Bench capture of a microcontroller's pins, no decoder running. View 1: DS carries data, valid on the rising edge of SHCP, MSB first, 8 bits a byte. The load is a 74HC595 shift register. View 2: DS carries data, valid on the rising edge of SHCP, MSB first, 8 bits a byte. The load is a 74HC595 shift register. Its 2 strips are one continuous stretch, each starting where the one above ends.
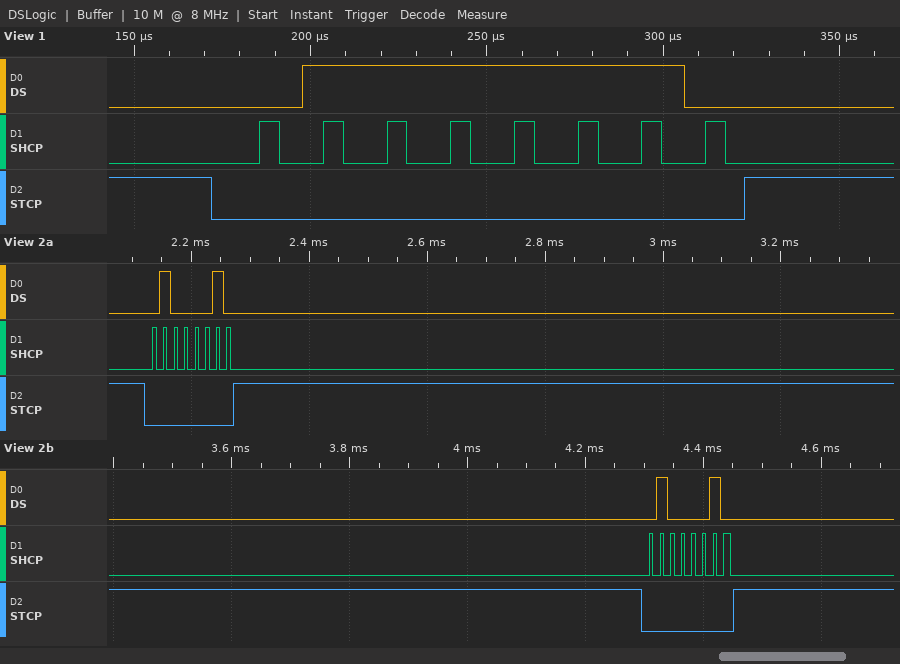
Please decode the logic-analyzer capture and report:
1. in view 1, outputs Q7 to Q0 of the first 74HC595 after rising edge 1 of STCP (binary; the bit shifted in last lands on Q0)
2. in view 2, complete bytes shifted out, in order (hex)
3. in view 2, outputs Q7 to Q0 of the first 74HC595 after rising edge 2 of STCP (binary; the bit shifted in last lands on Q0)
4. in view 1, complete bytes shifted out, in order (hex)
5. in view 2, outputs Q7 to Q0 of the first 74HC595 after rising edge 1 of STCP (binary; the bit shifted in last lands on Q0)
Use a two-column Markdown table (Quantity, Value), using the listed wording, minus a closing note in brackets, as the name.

| Quantity | Value |
|---|---|
| in view 1, outputs Q7 to Q0 of the first 74HC595 after rising edge 1 of STCP | 01111110 |
| in view 2, complete bytes shifted out, in order | 0x42 0x42 |
| in view 2, outputs Q7 to Q0 of the first 74HC595 after rising edge 2 of STCP | 01000010 |
| in view 1, complete bytes shifted out, in order | 0x7E |
| in view 2, outputs Q7 to Q0 of the first 74HC595 after rising edge 1 of STCP | 01000010 |
